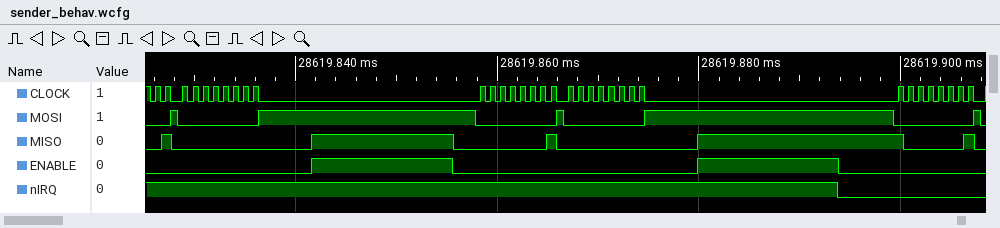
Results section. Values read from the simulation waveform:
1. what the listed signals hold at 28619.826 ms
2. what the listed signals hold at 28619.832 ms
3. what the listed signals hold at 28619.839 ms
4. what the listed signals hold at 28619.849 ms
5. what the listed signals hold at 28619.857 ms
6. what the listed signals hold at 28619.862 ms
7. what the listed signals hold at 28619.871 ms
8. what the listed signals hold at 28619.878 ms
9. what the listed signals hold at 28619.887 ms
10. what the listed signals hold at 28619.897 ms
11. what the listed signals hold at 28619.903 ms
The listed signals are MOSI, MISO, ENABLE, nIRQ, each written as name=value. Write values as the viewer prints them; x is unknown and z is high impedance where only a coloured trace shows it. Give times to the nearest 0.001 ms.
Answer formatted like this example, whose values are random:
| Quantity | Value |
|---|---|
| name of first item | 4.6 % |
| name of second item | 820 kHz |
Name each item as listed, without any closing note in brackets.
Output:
| Quantity | Value |
|---|---|
| what the listed signals hold at 28619.826 ms | MOSI=0, MISO=0, ENABLE=0, nIRQ=1 |
| what the listed signals hold at 28619.832 ms | MOSI=0, MISO=0, ENABLE=0, nIRQ=1 |
| what the listed signals hold at 28619.839 ms | MOSI=1, MISO=0, ENABLE=0, nIRQ=1 |
| what the listed signals hold at 28619.849 ms | MOSI=1, MISO=1, ENABLE=1, nIRQ=1 |
| what the listed signals hold at 28619.857 ms | MOSI=1, MISO=0, ENABLE=0, nIRQ=1 |
| what the listed signals hold at 28619.862 ms | MOSI=0, MISO=0, ENABLE=0, nIRQ=1 |
| what the listed signals hold at 28619.871 ms | MOSI=0, MISO=0, ENABLE=0, nIRQ=1 |
| what the listed signals hold at 28619.878 ms | MOSI=1, MISO=0, ENABLE=0, nIRQ=1 |
| what the listed signals hold at 28619.887 ms | MOSI=1, MISO=1, ENABLE=1, nIRQ=1 |
| what the listed signals hold at 28619.897 ms | MOSI=1, MISO=1, ENABLE=0, nIRQ=0 |
| what the listed signals hold at 28619.903 ms | MOSI=0, MISO=0, ENABLE=0, nIRQ=0 |
